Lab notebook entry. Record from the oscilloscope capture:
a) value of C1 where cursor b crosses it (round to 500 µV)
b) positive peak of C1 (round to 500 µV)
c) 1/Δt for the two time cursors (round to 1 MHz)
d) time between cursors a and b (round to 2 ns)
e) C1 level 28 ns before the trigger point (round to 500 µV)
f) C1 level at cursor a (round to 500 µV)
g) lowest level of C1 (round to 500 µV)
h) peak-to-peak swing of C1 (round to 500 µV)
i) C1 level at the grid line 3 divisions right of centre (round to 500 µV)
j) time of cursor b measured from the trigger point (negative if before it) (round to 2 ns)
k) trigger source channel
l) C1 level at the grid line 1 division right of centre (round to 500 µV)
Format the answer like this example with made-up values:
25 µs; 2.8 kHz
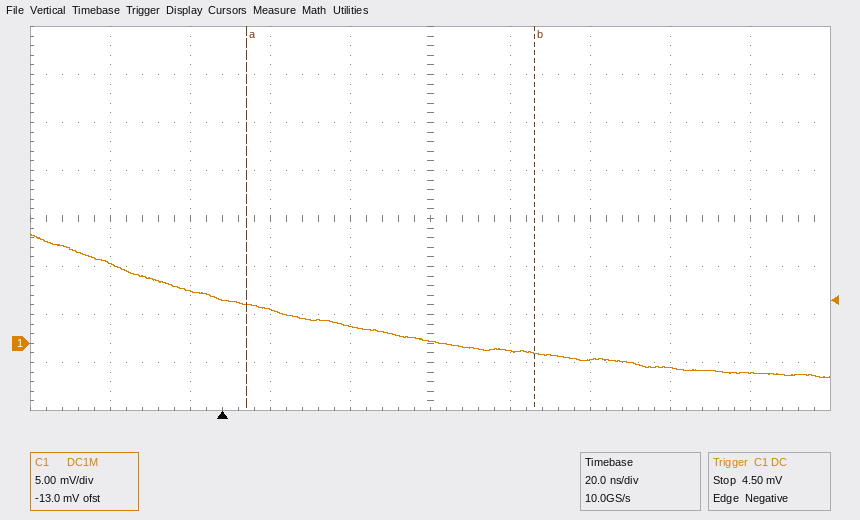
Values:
-1.0 mV; 11.5 mV; 14 MHz; 72 ns; 8.5 mV; 4.0 mV; -3.5 mV; 15.0 mV; -2.5 mV; +78 ns; C1; -1.0 mV
